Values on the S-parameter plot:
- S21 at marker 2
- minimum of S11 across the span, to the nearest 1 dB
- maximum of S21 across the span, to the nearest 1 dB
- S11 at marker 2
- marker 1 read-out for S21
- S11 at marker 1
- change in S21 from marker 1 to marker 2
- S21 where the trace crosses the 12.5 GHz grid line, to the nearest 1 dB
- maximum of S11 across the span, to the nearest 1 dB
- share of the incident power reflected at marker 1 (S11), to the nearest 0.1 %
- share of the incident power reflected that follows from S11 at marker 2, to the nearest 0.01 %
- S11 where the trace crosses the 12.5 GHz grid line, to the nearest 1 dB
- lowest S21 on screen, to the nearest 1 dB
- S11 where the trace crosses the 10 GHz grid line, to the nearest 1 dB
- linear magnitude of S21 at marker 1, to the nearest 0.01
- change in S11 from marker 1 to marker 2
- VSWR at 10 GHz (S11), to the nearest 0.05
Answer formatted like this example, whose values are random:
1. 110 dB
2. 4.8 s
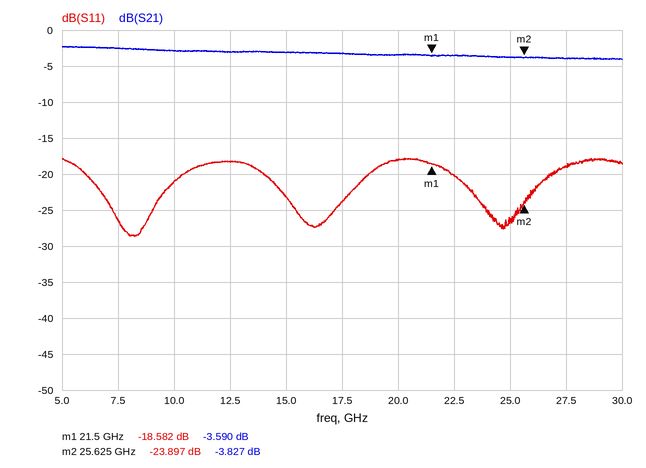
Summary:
1. -3.827 dB
2. -29 dB
3. -2 dB
4. -23.897 dB
5. -3.590 dB
6. -18.582 dB
7. -0.237 dB
8. -3 dB
9. -18 dB
10. 1.4 %
11. 0.41 %
12. -18 dB
13. -4 dB
14. -21 dB
15. 0.66
16. -5.315 dB
17. 1.20
